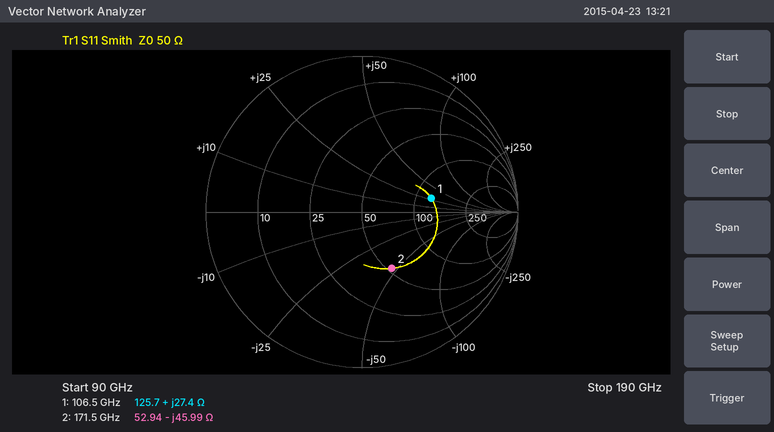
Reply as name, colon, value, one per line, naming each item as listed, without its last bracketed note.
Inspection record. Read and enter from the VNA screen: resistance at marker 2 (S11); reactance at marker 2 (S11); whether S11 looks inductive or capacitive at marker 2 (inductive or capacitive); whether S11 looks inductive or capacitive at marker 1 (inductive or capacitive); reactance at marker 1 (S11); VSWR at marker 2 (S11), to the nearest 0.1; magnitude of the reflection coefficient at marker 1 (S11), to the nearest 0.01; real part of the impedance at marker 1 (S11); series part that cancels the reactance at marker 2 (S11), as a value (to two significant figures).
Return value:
resistance at marker 2: 52.94 Ω
reactance at marker 2: -45.99 Ω
whether S11 looks inductive or capacitive at marker 2: capacitive
whether S11 looks inductive or capacitive at marker 1: inductive
reactance at marker 1: +27.4 Ω
VSWR at marker 2 (S11), to the nearest 0.1: 2.4
magnitude of the reflection coefficient at marker 1 (S11), to the nearest 0.01: 0.45
real part of the impedance at marker 1: 125.7 Ω
series part that cancels the reactance at marker 2 (S11), as a value: 43 pH
